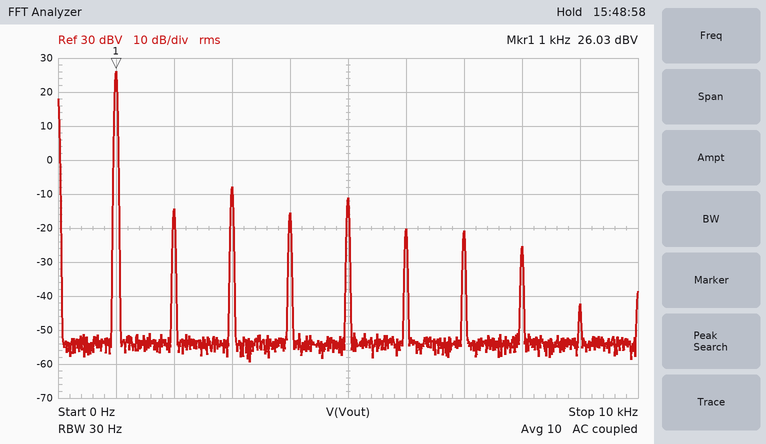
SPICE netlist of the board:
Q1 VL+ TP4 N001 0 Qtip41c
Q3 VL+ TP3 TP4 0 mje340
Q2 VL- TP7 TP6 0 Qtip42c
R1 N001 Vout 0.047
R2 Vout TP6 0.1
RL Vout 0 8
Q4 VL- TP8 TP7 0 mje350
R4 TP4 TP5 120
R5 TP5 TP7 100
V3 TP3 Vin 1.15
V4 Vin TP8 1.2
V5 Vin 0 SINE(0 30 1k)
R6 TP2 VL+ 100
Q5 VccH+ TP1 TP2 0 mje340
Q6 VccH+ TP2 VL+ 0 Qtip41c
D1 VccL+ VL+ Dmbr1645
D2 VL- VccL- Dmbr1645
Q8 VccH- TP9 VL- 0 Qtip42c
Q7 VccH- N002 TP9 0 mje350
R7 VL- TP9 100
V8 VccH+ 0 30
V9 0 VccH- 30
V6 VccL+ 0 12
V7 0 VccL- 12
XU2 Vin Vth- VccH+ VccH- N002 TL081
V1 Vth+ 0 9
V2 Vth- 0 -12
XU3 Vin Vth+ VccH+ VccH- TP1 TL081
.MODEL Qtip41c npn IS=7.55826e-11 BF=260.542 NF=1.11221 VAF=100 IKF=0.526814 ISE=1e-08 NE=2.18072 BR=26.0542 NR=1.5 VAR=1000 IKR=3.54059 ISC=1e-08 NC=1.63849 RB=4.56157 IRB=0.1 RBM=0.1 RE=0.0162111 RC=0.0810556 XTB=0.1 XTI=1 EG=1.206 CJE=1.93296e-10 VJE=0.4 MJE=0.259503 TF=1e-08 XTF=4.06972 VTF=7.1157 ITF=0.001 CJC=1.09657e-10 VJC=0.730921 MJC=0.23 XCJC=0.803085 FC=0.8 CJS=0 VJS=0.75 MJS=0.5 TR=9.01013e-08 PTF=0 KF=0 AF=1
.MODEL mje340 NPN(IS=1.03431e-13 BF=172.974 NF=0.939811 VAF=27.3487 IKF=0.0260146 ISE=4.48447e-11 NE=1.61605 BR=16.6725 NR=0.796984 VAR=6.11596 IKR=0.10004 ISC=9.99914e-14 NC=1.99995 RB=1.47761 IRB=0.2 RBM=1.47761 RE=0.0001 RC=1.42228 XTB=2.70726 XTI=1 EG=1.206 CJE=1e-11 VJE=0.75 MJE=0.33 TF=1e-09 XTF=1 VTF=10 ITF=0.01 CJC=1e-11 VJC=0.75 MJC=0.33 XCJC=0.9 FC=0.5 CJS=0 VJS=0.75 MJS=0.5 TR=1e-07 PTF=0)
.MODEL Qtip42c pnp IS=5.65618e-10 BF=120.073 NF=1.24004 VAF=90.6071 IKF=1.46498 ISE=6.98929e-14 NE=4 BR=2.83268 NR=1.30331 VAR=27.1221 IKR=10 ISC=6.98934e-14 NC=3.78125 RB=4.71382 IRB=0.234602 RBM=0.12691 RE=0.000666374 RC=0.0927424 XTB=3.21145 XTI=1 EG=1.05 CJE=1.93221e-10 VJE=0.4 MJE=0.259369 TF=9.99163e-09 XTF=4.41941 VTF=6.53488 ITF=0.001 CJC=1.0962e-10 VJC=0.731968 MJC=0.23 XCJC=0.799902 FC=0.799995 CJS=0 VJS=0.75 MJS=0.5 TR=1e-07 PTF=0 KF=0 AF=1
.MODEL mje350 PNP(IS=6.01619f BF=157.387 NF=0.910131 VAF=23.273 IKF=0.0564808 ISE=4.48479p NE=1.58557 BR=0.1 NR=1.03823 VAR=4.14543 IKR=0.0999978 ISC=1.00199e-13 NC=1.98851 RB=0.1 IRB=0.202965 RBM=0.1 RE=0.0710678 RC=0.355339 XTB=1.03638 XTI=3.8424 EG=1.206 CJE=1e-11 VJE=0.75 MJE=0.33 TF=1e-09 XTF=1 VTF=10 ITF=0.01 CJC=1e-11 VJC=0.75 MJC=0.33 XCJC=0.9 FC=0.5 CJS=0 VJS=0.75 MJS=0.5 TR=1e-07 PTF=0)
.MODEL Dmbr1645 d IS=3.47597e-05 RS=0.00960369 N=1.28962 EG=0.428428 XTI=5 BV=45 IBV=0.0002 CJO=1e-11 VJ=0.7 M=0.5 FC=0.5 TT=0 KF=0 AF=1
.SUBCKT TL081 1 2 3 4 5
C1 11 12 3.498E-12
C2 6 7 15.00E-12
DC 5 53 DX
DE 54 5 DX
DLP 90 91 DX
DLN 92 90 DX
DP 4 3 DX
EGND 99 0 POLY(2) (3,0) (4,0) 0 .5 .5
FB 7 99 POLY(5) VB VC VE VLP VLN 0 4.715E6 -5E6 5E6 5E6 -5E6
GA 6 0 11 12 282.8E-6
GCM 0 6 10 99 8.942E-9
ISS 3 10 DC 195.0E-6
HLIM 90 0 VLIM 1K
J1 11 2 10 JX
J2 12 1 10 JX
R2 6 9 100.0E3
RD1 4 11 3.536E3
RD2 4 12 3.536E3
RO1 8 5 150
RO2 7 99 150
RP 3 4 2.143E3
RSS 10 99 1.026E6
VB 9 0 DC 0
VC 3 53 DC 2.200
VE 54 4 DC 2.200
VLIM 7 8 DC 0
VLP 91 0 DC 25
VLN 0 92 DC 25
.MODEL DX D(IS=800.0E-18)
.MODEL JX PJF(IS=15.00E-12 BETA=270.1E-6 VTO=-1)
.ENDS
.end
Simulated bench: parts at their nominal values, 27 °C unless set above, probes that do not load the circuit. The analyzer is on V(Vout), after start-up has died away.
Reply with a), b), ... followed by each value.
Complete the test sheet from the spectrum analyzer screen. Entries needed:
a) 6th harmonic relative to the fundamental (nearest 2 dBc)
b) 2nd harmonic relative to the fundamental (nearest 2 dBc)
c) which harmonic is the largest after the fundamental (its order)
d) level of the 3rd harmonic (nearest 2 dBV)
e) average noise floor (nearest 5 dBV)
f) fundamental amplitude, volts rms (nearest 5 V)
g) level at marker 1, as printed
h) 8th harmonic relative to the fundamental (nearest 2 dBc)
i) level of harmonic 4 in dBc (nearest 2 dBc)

a) -46 dBc
b) -40 dBc
c) 3
d) -8 dBV
e) -55 dBV
f) 20 V
g) 26.03 dBV
h) -52 dBc
i) -42 dBc
